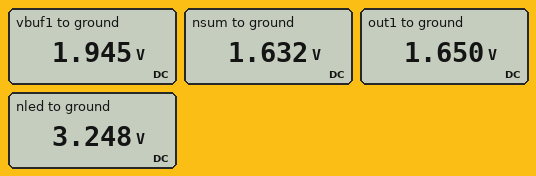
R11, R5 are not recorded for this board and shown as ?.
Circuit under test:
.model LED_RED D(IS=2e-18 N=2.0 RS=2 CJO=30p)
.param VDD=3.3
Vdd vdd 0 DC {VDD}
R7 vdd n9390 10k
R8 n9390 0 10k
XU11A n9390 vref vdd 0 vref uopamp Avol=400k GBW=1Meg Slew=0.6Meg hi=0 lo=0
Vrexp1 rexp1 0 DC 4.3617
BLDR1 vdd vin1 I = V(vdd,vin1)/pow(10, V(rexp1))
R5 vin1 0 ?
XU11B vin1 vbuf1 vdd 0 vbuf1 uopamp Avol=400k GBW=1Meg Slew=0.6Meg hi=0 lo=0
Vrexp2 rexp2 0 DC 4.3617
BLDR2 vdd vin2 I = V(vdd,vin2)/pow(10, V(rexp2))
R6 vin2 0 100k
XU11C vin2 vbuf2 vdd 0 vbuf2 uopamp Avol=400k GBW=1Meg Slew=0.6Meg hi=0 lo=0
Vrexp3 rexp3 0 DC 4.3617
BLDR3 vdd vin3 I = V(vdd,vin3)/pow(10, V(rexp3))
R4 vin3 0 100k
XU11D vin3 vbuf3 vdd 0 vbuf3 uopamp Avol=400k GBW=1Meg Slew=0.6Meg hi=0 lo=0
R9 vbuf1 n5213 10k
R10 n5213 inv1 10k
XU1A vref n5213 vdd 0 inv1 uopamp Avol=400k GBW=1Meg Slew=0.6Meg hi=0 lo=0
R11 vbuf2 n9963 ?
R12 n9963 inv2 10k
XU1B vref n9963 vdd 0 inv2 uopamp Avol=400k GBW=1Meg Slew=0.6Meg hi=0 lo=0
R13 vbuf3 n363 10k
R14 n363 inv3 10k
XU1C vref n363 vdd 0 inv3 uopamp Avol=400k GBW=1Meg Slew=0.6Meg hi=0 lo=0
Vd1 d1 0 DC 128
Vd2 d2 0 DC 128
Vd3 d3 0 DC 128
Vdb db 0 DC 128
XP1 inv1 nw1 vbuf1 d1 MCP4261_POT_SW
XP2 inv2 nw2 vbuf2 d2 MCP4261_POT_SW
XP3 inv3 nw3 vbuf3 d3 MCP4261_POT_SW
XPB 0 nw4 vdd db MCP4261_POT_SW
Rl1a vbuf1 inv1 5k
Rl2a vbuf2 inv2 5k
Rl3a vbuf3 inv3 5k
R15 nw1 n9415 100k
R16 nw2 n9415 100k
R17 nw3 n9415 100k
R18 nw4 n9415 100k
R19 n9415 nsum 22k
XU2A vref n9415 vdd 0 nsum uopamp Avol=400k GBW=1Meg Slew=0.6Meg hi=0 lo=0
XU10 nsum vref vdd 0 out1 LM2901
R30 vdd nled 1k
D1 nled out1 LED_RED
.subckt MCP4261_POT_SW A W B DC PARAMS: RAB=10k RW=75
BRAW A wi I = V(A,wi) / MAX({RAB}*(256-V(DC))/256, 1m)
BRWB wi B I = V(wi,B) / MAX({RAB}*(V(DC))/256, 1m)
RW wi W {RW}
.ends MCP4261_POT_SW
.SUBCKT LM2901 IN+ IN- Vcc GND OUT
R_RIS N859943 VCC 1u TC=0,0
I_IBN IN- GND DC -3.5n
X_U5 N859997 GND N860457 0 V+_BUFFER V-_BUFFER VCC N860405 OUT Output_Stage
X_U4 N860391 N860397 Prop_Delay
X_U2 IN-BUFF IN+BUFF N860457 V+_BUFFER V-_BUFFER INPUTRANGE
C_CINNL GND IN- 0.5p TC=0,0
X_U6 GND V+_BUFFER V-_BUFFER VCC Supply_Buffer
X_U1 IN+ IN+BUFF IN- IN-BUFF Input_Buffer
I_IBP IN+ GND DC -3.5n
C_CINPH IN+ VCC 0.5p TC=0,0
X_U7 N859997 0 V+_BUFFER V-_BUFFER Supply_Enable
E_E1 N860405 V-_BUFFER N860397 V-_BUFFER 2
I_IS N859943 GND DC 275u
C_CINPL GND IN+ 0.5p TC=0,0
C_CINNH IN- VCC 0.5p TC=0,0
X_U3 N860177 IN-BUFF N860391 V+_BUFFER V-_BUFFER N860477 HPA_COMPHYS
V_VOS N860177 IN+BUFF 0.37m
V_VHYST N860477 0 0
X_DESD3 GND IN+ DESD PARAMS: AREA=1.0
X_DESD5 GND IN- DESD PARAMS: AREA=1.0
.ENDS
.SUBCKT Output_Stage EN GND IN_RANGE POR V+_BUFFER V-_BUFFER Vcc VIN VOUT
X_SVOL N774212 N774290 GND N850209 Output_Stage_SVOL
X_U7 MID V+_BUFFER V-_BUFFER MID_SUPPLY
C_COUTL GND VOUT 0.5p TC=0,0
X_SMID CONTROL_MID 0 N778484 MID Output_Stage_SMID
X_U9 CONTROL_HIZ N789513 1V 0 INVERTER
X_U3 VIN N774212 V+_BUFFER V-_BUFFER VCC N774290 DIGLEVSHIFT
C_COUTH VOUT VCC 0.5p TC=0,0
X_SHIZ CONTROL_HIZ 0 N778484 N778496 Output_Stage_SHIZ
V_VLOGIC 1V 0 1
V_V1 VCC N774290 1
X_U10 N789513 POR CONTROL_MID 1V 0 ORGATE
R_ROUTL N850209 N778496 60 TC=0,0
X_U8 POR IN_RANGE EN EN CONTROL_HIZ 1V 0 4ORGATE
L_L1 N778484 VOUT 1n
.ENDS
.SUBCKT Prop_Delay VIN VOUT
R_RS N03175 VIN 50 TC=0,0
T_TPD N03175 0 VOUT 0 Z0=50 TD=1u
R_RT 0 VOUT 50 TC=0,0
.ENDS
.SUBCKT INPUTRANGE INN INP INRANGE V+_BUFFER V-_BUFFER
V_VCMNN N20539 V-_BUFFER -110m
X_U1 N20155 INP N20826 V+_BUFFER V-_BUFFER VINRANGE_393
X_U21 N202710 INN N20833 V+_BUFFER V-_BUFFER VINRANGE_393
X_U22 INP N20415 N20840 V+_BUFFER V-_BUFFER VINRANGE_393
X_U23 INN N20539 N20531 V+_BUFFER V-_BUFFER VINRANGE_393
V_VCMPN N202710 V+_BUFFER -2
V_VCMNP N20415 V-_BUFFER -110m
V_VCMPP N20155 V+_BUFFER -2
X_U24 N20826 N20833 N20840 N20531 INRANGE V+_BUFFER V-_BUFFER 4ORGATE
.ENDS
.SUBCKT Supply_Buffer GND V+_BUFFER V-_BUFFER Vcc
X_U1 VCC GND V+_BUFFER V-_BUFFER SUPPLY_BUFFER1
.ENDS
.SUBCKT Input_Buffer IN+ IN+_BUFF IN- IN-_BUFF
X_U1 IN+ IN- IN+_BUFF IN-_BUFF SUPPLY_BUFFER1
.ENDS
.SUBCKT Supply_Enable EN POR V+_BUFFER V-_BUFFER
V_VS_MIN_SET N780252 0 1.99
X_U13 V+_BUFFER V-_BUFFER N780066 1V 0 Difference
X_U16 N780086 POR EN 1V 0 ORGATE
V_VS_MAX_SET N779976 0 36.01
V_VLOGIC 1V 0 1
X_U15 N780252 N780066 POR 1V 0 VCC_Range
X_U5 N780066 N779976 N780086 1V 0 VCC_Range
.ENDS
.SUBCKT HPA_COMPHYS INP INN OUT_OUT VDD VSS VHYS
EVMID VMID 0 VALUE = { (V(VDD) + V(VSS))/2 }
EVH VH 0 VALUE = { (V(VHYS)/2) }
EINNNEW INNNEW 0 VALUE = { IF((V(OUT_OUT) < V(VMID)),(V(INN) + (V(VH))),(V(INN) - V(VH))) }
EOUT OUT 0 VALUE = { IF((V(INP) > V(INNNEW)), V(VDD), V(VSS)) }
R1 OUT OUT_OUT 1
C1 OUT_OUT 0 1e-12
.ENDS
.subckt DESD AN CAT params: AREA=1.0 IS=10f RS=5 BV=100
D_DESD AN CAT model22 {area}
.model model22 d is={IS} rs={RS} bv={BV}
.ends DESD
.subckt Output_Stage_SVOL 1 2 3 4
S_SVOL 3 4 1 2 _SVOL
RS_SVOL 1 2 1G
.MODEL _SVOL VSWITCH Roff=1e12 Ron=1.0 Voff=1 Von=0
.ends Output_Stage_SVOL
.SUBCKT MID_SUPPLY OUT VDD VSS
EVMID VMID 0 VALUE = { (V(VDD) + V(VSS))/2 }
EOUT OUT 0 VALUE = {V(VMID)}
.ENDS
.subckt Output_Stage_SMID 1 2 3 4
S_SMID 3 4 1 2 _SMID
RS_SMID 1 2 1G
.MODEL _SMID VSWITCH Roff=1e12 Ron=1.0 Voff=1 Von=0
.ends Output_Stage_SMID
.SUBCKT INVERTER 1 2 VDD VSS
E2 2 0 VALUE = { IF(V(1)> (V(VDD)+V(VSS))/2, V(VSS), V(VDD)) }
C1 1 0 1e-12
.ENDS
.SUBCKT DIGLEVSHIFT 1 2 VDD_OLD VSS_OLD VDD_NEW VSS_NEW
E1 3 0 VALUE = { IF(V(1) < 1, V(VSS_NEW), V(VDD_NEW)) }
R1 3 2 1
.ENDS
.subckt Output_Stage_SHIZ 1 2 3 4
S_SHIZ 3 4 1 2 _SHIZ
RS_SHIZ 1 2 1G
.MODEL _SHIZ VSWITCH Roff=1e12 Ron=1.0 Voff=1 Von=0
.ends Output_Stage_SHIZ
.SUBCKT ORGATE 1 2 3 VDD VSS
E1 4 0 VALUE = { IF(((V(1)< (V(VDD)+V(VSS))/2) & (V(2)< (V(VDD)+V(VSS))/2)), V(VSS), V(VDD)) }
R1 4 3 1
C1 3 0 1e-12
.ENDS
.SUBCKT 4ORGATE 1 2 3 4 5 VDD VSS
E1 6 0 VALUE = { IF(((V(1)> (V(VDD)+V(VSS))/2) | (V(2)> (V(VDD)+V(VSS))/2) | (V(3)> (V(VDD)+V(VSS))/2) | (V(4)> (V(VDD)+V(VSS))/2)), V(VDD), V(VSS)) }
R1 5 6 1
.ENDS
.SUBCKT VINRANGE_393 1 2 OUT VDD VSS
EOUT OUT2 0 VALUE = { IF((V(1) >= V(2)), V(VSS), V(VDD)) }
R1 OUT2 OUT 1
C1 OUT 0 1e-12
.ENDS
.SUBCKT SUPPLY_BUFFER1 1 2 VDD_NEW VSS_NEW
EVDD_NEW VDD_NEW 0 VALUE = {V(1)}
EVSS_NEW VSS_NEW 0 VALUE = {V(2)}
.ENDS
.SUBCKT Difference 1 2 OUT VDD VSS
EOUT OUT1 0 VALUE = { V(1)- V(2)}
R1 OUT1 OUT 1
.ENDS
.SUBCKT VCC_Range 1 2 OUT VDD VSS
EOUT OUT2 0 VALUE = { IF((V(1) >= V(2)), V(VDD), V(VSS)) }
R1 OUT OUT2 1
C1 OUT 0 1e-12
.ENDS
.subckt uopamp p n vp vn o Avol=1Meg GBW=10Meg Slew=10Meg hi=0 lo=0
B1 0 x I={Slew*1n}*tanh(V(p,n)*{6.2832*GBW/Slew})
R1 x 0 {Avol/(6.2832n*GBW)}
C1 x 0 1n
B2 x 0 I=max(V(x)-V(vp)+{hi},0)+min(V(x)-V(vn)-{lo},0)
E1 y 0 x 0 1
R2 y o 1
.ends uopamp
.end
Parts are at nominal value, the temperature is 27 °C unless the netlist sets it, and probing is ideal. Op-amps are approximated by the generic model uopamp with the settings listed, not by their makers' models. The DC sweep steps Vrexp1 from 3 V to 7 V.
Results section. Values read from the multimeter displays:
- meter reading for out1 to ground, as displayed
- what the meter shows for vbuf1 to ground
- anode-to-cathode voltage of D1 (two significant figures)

1.650 V
1.945 V
1.6 V
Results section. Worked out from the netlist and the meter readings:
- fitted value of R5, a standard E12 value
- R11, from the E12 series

33 kΩ
12 kΩ
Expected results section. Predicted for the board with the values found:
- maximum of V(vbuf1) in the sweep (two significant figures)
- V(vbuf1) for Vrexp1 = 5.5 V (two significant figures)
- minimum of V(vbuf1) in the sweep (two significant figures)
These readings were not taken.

3.2 V
310 mV
11 mV
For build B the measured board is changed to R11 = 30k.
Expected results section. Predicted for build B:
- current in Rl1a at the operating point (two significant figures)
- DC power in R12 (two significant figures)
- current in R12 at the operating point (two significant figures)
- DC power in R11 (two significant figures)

120 µA
12 µW
34 µA
36 µW
